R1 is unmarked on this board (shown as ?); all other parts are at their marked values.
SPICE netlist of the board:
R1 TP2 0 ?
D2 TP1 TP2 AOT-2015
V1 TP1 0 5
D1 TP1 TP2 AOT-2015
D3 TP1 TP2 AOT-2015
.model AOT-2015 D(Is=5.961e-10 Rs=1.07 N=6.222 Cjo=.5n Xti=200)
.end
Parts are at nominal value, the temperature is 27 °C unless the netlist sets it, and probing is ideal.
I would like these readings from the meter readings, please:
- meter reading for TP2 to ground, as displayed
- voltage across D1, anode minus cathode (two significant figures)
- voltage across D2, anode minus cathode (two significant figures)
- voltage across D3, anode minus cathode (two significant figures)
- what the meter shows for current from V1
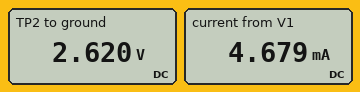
2.620 V
2.4 V
2.4 V
2.4 V
4.679 mA
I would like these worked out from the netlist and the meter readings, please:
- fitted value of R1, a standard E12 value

560 Ω
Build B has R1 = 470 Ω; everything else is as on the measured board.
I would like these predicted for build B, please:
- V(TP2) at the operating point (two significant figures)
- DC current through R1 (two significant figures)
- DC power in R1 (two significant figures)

2.6 V
5.5 mA
14 mW
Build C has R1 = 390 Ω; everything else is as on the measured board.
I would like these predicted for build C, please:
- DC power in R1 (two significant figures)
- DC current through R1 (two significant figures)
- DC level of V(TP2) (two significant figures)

17 mW
6.6 mA
2.6 V
